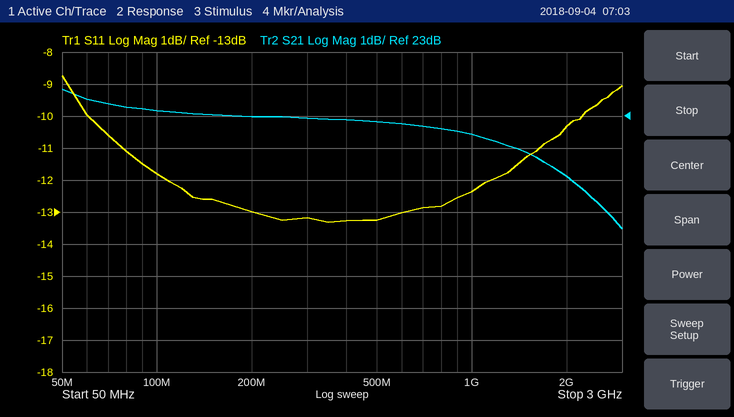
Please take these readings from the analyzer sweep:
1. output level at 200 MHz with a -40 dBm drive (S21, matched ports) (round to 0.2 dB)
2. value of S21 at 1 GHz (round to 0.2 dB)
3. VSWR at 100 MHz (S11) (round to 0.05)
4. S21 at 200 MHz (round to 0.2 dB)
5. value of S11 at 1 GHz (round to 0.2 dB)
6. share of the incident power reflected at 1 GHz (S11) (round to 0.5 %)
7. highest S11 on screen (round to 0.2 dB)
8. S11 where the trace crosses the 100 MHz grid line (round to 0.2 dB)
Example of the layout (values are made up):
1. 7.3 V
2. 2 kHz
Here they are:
1. -17.0 dBm
2. 22.4 dB
3. 1.70
4. 23.0 dB
5. -12.4 dB
6. 6.0 %
7. -8.8 dB
8. -11.8 dB
